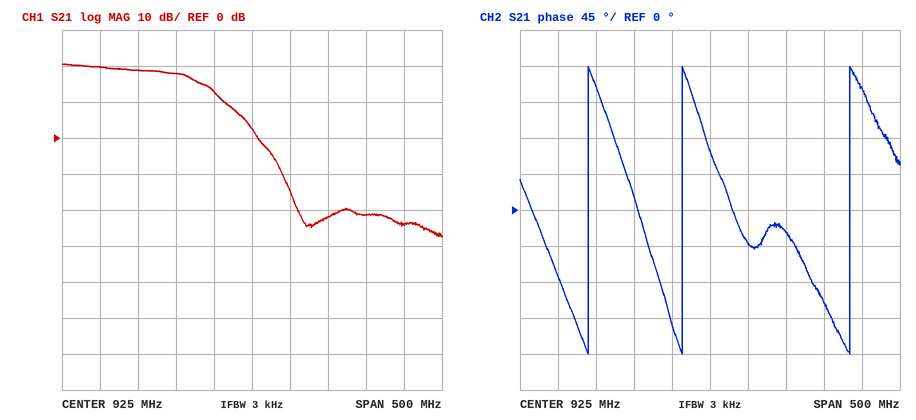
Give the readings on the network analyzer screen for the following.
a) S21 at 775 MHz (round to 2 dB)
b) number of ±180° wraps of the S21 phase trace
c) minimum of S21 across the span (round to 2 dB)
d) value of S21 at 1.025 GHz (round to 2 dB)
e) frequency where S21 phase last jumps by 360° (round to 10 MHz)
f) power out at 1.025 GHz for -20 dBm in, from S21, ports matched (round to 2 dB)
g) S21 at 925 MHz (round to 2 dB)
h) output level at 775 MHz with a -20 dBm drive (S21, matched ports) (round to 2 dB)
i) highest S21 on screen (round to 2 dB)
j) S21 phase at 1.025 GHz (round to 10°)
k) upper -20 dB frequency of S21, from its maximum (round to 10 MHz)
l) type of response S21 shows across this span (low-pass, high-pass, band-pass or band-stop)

18 dB
3
-28 dB
-22 dB
1.11 GHz
-42 dBm
2 dB
-2 dBm
20 dB
-30°
930 MHz
low-pass
